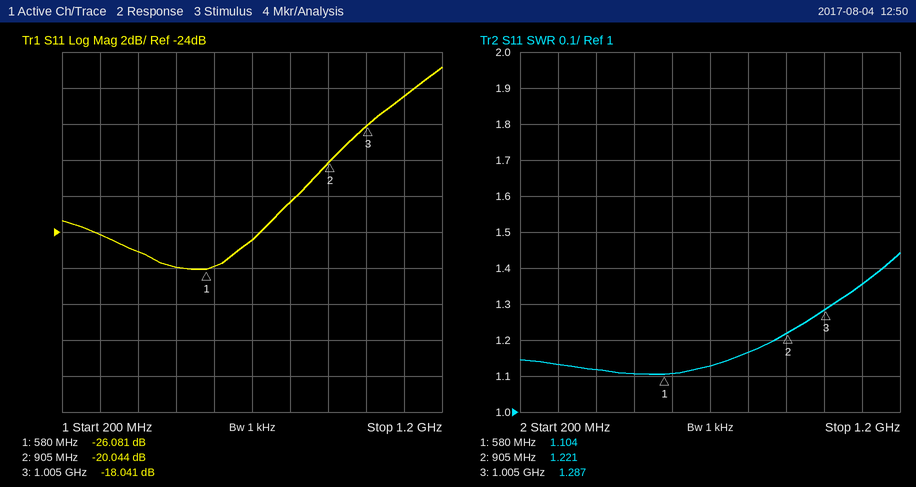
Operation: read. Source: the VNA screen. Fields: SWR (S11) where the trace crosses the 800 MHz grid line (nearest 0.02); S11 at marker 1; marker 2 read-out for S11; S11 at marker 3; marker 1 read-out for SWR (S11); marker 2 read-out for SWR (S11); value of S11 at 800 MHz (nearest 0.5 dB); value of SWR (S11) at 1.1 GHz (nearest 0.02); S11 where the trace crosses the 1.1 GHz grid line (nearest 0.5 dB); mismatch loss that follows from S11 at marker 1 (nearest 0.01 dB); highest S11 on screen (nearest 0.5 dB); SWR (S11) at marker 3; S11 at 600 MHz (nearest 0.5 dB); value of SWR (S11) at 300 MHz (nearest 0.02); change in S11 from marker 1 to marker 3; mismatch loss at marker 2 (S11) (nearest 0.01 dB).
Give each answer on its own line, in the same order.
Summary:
1.16
-26.081 dB
-20.044 dB
-18.041 dB
1.104
1.221
-22.5 dB
1.36
-16.5 dB
0.01 dB
-15.0 dB
1.287
-26.0 dB
1.14
8.040 dB
0.04 dB
